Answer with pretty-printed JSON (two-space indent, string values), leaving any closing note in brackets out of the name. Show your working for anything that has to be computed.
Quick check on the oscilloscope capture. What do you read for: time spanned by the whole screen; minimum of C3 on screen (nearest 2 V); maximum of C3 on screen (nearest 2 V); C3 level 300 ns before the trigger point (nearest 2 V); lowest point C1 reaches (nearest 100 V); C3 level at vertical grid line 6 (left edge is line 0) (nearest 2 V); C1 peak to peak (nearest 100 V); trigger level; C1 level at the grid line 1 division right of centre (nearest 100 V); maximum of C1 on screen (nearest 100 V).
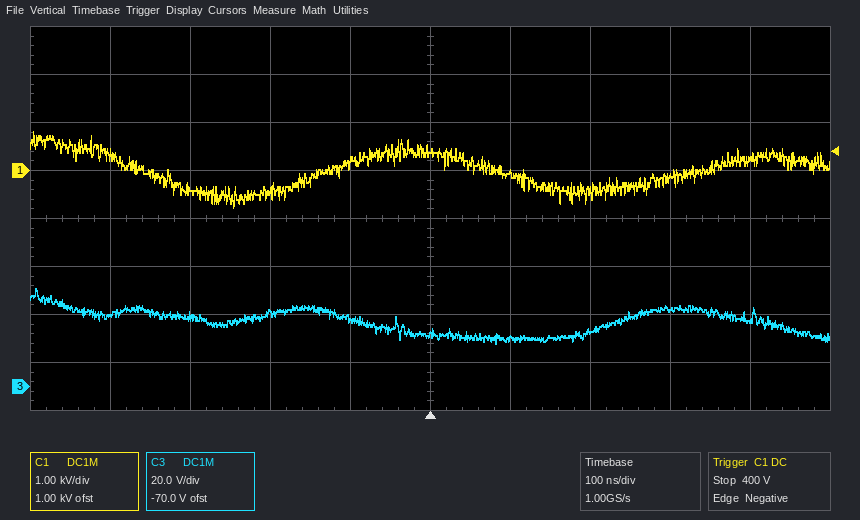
{
  "time spanned by the whole screen": "1 µs",
  "minimum of C3 on screen": "18 V",
  "maximum of C3 on screen": "40 V",
  "C3 level 300 ns before the trigger point": "30 V",
  "lowest point C1 reaches": "-800 V",
  "C3 level at vertical grid line 6 (left edge is line 0)": "20 V",
  "C1 peak to peak": "800 V − (-800 V) = 1.6 kV",
  "trigger level": "400 V",
  "C1 level at the grid line 1 division right of centre": "-100 V",
  "maximum of C1 on screen": "800 V"
}
